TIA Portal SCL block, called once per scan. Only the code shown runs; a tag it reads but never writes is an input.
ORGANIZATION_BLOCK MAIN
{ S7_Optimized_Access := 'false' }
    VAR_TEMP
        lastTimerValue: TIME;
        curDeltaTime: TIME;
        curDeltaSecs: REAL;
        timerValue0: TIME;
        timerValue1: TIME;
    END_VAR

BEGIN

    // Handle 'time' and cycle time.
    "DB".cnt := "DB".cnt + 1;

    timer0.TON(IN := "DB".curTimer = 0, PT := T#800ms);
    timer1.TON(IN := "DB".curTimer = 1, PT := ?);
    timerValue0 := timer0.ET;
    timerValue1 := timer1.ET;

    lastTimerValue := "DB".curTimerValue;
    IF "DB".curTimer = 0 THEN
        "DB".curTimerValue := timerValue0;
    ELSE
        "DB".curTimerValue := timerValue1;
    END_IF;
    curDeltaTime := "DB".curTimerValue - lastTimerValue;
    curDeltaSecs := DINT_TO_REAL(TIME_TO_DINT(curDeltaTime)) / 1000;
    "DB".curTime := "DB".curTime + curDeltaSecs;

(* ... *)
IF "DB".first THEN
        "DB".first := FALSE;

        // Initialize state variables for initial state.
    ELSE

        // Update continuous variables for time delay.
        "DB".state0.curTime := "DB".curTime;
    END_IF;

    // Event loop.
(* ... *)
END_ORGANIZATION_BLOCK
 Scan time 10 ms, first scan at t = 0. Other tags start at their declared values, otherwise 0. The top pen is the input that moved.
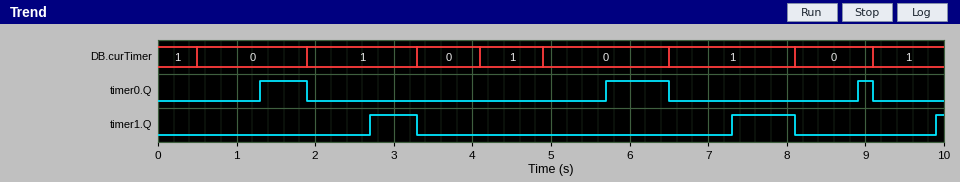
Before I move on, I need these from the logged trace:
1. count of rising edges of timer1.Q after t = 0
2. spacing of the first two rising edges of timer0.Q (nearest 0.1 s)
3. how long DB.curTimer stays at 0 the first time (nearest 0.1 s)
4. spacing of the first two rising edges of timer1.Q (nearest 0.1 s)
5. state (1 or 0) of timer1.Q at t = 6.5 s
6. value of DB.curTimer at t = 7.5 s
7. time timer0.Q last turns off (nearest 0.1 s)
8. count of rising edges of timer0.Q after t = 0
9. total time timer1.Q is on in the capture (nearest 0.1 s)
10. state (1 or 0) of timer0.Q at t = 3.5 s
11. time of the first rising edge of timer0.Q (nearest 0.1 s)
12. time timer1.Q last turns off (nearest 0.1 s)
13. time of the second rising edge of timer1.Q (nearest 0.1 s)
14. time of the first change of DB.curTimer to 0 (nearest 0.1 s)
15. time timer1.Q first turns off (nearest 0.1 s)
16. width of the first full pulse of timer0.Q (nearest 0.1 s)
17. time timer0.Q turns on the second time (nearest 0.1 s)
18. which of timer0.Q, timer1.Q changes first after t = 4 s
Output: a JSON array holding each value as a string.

["3", "4.4 s", "1.4 s", "4.6 s", "0", "1", "9.1 s", "3", "1.5 s", "0", "1.3 s", "8.1 s", "7.3 s", "0.5 s", "3.3 s", "0.6 s", "5.7 s", "timer0.Q"]
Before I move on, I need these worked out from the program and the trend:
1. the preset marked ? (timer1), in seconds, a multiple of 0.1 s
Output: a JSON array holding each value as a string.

["0.8 s"]
